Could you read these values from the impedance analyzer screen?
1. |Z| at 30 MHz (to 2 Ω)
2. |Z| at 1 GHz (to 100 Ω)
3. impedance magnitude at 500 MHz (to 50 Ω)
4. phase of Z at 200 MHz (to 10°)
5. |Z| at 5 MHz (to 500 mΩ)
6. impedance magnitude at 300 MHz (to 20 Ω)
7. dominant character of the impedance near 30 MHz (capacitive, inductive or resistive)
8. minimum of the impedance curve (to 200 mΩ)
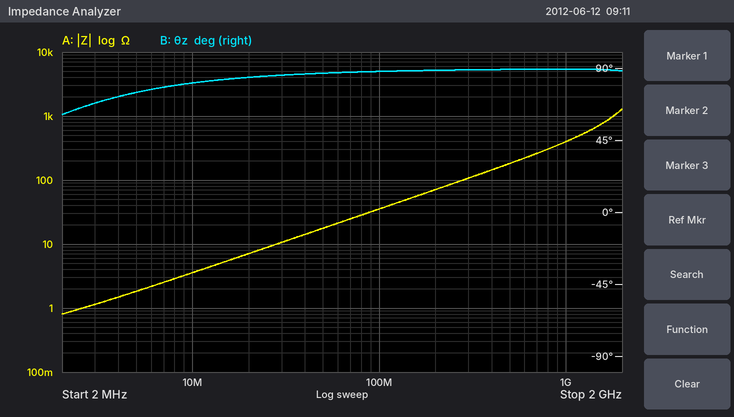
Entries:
10 Ω
400 Ω
200 Ω
90°
2.0 Ω
100 Ω
inductive
800 mΩ
